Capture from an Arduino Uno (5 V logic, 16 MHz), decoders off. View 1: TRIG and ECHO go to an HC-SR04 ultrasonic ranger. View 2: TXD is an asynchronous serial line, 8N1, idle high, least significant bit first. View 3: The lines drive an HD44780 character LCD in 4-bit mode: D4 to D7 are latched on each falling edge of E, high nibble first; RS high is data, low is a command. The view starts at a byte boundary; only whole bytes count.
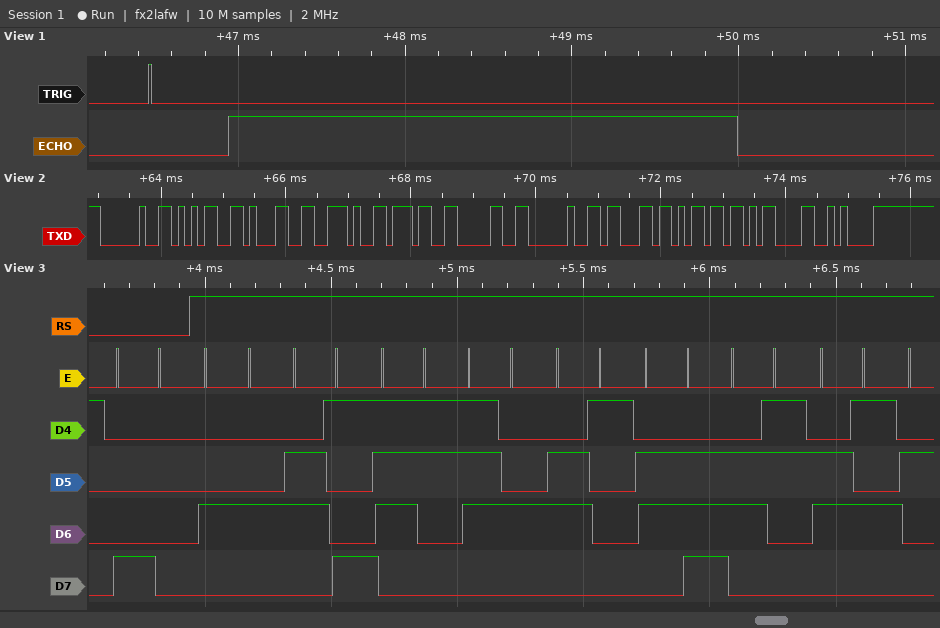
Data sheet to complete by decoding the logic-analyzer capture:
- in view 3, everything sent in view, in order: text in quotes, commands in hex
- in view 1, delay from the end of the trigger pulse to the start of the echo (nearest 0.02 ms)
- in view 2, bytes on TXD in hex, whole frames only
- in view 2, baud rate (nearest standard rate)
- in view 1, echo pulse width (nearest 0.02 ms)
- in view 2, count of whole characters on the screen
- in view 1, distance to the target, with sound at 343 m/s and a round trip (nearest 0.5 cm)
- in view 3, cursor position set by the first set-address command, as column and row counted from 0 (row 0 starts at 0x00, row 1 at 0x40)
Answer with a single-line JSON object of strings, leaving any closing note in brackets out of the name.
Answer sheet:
{"in view 3, everything sent in view, in order: text in quotes, commands in hex": "0x80 \"Distance\"", "in view 1, delay from the end of the trigger pulse to the start of the echo": "0.46 ms", "in view 2, bytes on TXD in hex, whole frames only": "0x20 0x35 0x31 0x2E 0x37 0x30 0x20 0x63 0x6D 0x0D 0x0A", "in view 2, baud rate": "9600 baud", "in view 1, echo pulse width": "3.06 ms", "in view 2, count of whole characters on the screen": "11", "in view 1, distance to the target, with sound at 343 m/s and a round trip": "52.5 cm", "in view 3, cursor position set by the first set-address command, as column and row counted from 0": "column 0, row 0"}
